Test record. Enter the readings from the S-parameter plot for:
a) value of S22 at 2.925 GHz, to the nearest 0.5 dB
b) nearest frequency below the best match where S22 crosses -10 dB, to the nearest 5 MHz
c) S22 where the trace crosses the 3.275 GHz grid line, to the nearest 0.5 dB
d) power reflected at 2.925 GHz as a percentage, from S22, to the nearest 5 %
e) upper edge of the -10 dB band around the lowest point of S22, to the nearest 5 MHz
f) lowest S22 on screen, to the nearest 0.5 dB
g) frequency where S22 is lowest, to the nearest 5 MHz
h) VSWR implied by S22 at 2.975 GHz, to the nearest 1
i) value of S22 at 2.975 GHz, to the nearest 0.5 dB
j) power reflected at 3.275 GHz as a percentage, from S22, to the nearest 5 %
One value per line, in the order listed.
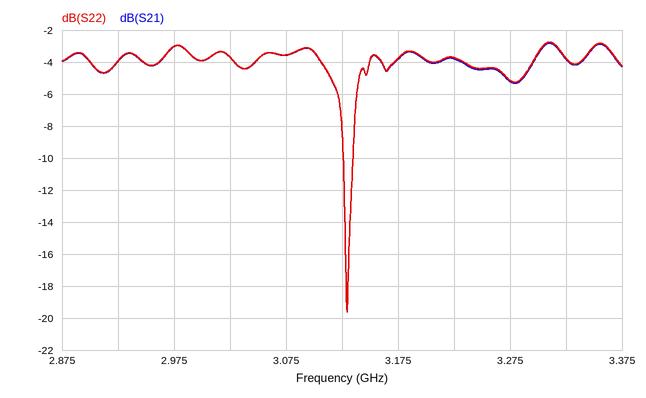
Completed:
-4.0 dB
3.125 GHz
-5.0 dB
40 %
3.135 GHz
-19.5 dB
3.130 GHz
6
-3.0 dB
30 %
